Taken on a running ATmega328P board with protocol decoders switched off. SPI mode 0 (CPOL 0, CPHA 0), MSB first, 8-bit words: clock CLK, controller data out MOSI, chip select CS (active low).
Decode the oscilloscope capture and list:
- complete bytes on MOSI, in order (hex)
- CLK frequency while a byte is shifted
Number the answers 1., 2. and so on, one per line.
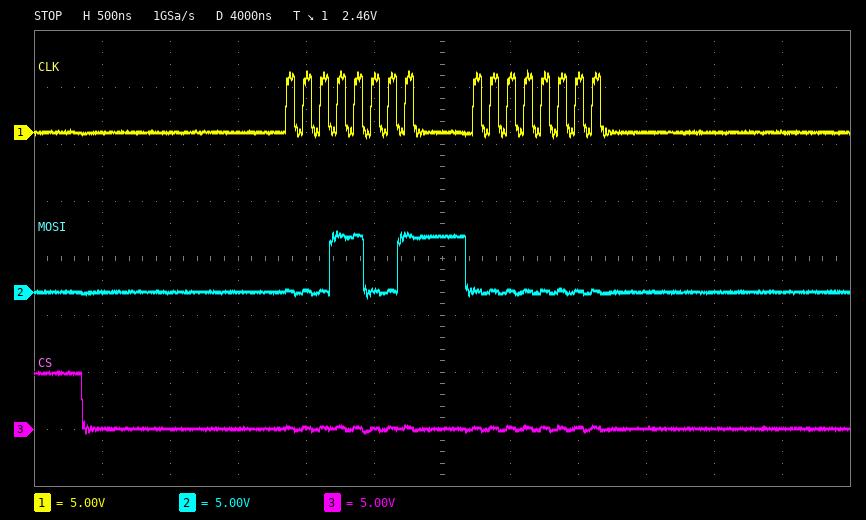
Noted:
1. 19 00
2. 8 MHz
